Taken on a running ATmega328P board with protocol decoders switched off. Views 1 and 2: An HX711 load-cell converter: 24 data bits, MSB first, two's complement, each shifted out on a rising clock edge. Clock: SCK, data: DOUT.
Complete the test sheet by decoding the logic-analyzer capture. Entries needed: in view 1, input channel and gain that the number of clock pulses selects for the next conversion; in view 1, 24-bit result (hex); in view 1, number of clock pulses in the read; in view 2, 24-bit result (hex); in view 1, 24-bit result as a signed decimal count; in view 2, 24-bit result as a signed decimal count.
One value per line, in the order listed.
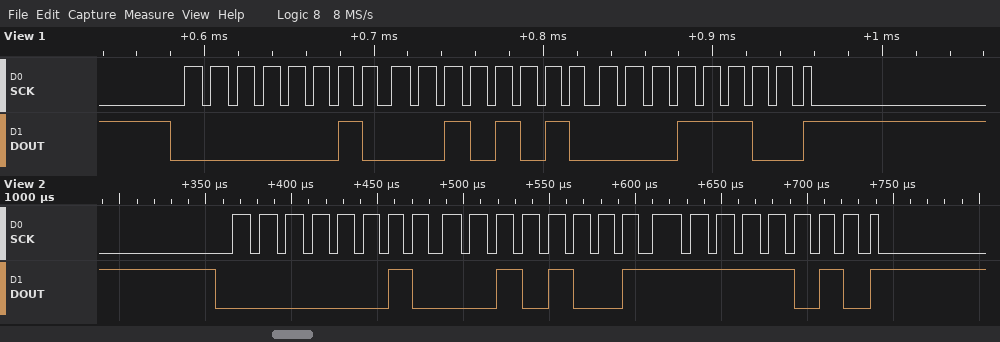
channel A, gain 128
0x022A1C
25
0x0229FA
141852
141818
